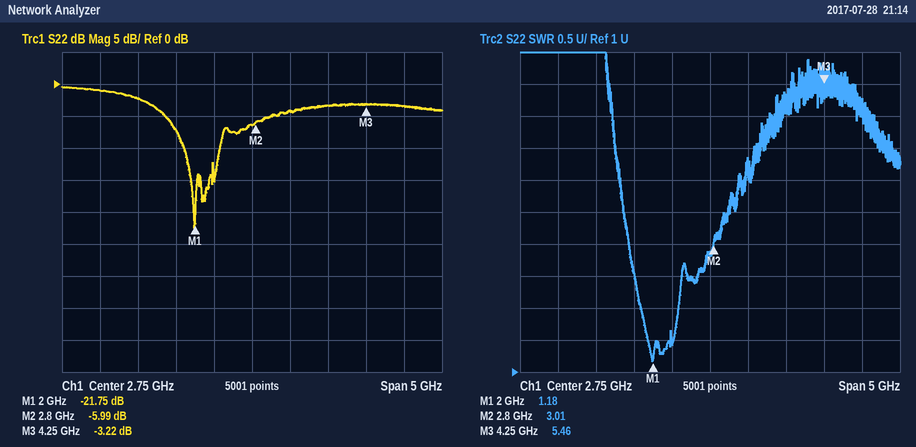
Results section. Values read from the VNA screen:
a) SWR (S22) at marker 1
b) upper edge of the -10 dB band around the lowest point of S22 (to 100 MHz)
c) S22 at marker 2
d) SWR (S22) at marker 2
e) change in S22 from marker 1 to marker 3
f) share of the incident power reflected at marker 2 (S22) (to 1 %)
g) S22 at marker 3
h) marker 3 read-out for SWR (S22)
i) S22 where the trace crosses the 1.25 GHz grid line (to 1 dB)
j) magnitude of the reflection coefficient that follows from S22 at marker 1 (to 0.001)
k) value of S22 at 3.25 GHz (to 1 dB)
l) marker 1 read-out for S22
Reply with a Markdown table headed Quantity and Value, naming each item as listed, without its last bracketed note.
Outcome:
| Quantity | Value |
|---|---|
| SWR (S22) at marker 1 | 1.18 |
| upper edge of the -10 dB band around the lowest point of S22 | 2.3 GHz |
| S22 at marker 2 | -5.99 dB |
| SWR (S22) at marker 2 | 3.01 |
| change in S22 from marker 1 to marker 3 | 18.53 dB |
| share of the incident power reflected at marker 2 (S22) | 25 % |
| S22 at marker 3 | -3.22 dB |
| marker 3 read-out for SWR | 5.46 |
| S22 where the trace crosses the 1.25 GHz grid line | -2 dB |
| magnitude of the reflection coefficient that follows from S22 at marker 1 | 0.082 |
| value of S22 at 3.25 GHz | -4 dB |
| marker 1 read-out for S22 | -21.75 dB |
